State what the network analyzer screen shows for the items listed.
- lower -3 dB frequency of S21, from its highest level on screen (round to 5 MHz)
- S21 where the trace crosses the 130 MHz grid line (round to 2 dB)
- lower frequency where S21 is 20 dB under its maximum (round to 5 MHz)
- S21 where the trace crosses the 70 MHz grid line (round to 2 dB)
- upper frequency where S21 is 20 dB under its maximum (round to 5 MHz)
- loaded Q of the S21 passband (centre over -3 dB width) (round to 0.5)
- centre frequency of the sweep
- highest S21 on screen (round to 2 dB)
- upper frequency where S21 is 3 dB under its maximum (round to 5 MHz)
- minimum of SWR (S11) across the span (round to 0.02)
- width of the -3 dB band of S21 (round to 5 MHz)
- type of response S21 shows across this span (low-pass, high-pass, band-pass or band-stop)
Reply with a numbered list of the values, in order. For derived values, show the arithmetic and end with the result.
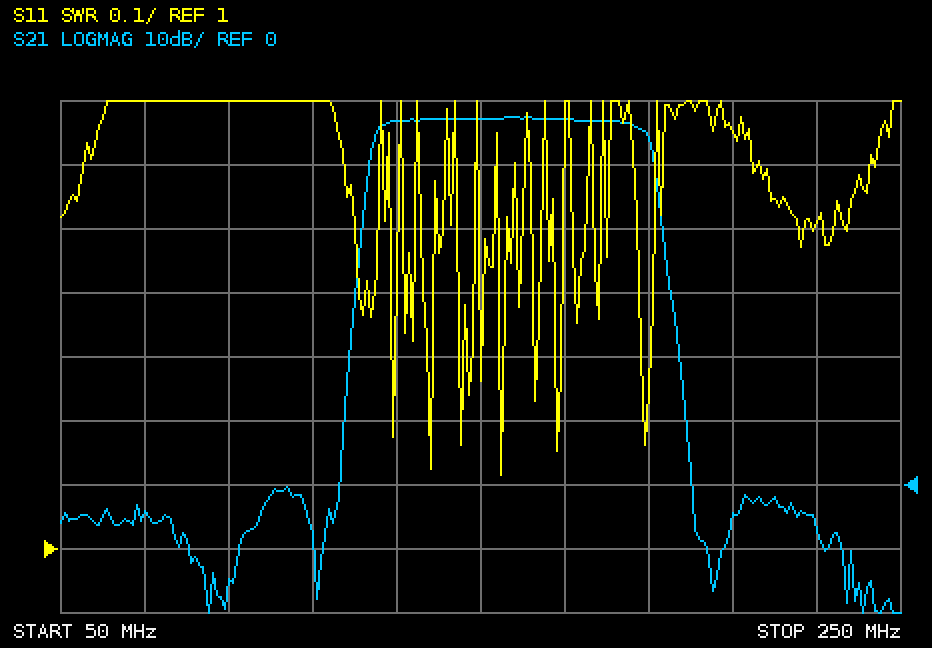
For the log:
1. 125 MHz
2. 56 dB
3. 120 MHz
4. -4 dB
5. 195 MHz
6. 157.5 MHz / 65 MHz ≈ 2.42, so 2.5 to the nearest 0.5
7. 150 MHz
8. 58 dB
9. 190 MHz
10. 1.12
11. 190 MHz − 125 MHz = 65 MHz
12. band-pass
